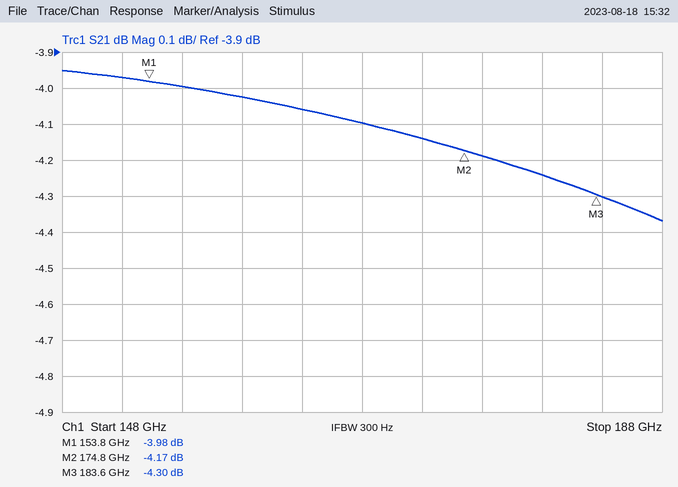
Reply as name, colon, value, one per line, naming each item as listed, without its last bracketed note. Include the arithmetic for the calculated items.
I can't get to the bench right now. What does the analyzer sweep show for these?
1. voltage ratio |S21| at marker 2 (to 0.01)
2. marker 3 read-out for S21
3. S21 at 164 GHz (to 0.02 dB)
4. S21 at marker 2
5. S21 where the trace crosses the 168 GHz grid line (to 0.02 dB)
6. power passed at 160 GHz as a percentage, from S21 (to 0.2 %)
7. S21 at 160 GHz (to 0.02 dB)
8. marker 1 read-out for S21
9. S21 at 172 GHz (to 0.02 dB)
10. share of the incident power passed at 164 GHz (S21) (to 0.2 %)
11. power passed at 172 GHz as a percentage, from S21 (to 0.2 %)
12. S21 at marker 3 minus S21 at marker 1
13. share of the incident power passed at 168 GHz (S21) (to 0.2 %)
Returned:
voltage ratio |S21| at marker 2: 10^(-4.17/20) ≈ 0.62
marker 3 read-out for S21: -4.30 dB
S21 at 164 GHz: -4.06 dB
S21 at marker 2: -4.17 dB
S21 where the trace crosses the 168 GHz grid line: -4.10 dB
power passed at 160 GHz as a percentage, from S21: 10^(-4.02/10) ≈ 39.6 %
S21 at 160 GHz: -4.02 dB
marker 1 read-out for S21: -3.98 dB
S21 at 172 GHz: -4.14 dB
share of the incident power passed at 164 GHz (S21): 10^(-4.06/10) ≈ 39.3 %, so 39.2 % to the nearest 0.2 %
power passed at 172 GHz as a percentage, from S21: 10^(-4.14/10) ≈ 38.5 %, so 38.6 % to the nearest 0.2 %
S21 at marker 3 minus S21 at marker 1: -4.3 − (-3.98) = -0.32 dB
share of the incident power passed at 168 GHz (S21): 10^(-4.1/10) ≈ 38.9 %, so 39.0 % to the nearest 0.2 %
